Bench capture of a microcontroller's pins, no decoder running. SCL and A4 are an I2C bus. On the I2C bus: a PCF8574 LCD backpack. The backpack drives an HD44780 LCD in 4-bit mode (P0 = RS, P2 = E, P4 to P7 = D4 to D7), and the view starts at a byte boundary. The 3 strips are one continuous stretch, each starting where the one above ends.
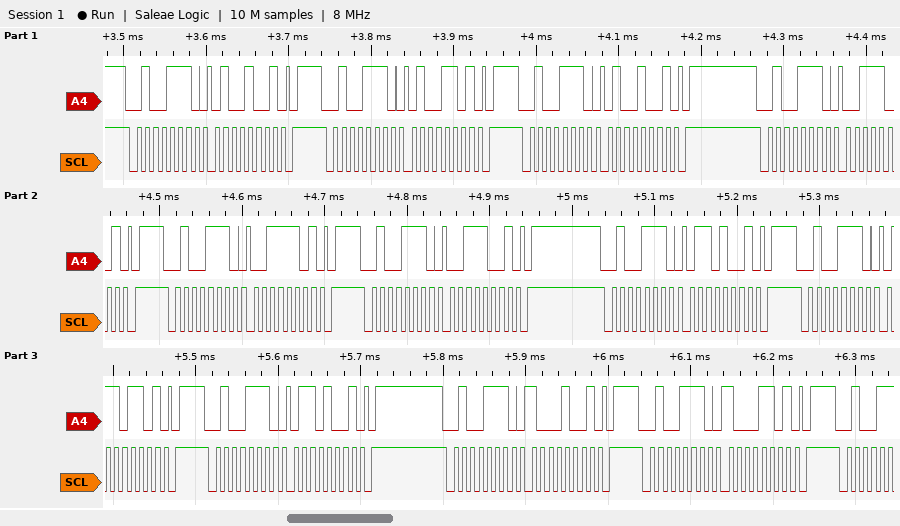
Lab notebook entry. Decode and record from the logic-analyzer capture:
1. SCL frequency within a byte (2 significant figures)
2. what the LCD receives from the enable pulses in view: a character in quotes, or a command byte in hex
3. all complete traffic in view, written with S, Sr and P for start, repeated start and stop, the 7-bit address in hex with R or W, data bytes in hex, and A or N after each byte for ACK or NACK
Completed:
100 kHz
'C'
S 27W A 49 A P S 27W A 4D A P S 27W A 49 A P S 27W A 39 A P S 27W A 3D A P S 27W A 39 A P S 27W A 69 A P S 27W A 6D A P S 27W A 69 A P S 27W A 89 A P S 27W A 8D A P
